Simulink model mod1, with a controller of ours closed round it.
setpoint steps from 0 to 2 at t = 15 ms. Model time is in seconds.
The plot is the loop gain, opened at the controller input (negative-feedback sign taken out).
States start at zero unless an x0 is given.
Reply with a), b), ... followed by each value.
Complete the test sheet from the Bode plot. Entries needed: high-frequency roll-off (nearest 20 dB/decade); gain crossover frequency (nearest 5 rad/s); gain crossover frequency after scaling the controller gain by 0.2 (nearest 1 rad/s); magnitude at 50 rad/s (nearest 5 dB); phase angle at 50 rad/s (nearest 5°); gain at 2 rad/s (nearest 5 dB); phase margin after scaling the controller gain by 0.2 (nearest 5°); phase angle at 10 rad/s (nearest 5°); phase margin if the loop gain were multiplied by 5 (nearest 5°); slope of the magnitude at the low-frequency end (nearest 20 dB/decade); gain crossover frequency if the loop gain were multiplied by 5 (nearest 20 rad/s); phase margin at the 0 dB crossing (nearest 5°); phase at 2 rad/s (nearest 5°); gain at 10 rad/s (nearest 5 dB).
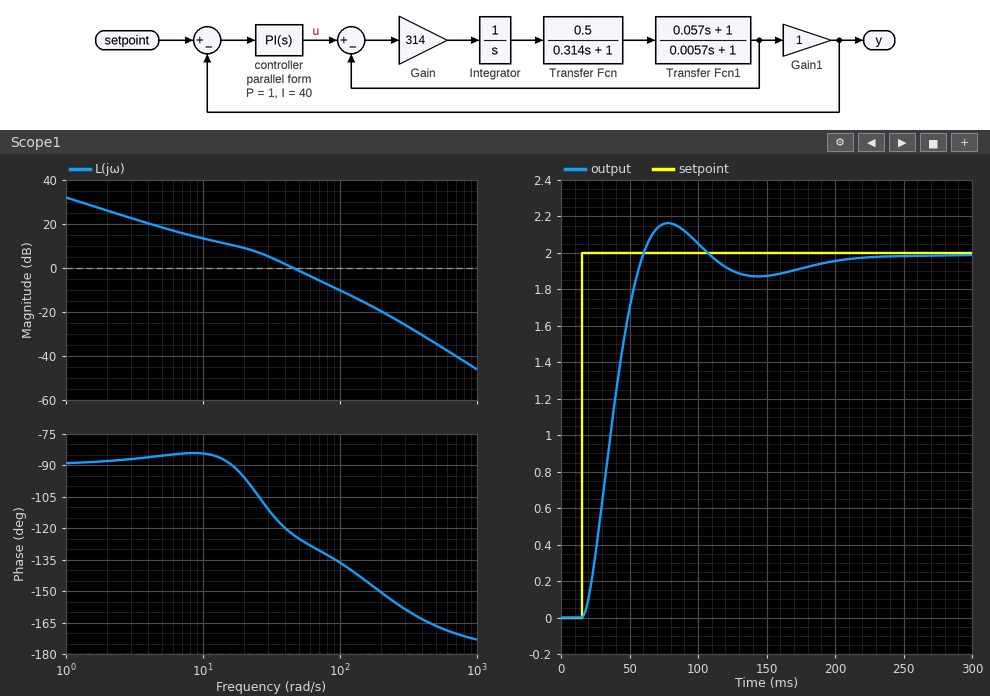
a) -40 dB/decade
b) 45 rad/s
c) 9 rad/s
d) 0 dB
e) -125°
f) 25 dB
g) 95°
h) -85°
i) 40°
j) -20 dB/decade
k) 140 rad/s
l) 55°
m) -90°
n) 15 dB
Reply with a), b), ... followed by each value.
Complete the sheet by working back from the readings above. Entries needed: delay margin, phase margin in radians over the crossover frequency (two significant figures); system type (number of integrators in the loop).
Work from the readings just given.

a) 0.021 s
b) 1
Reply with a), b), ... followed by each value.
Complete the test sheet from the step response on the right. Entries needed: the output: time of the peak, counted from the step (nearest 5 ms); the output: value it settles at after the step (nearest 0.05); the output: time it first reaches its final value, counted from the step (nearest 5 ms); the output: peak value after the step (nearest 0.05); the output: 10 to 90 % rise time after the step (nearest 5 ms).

a) 65 ms
b) 2.00
c) 45 ms
d) 2.15
e) 30 ms
